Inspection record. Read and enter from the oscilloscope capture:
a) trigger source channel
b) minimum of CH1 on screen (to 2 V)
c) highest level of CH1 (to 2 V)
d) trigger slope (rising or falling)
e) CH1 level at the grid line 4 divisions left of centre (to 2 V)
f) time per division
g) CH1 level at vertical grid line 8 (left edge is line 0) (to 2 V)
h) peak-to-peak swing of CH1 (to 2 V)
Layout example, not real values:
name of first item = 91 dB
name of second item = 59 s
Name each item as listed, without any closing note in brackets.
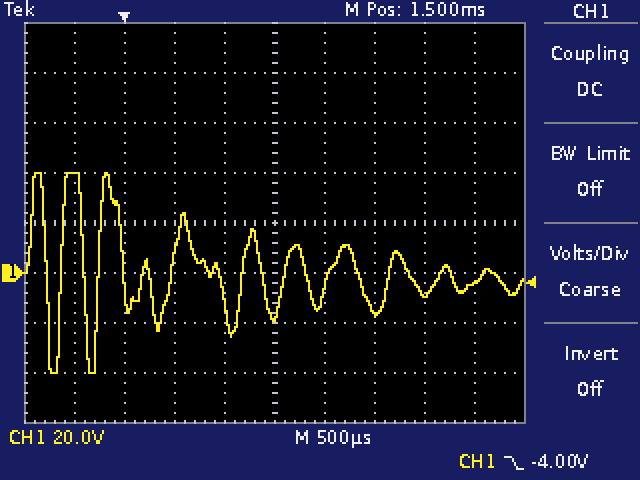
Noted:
trigger source channel = CH1
minimum of CH1 on screen = -40 V
highest level of CH1 = 40 V
trigger slope = falling
CH1 level at the grid line 4 divisions left of centre = 40 V
time per division = 500 µs
CH1 level at vertical grid line 8 (left edge is line 0) = -8 V
peak-to-peak swing of CH1 = 80 V
